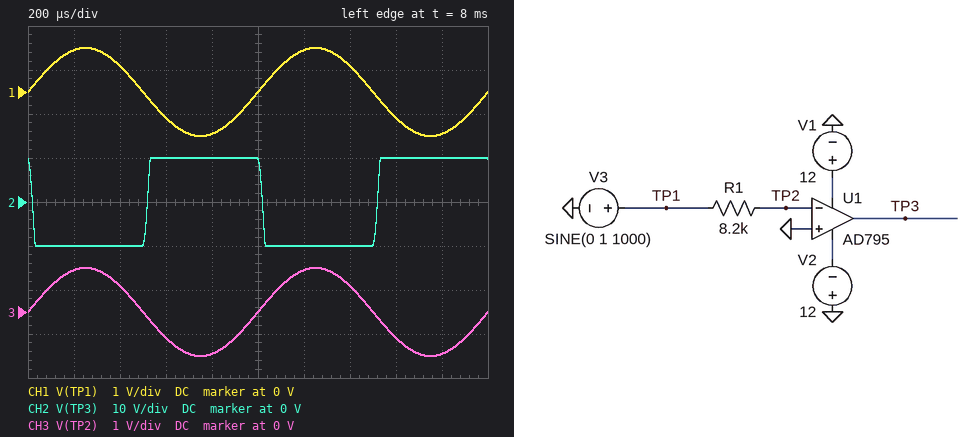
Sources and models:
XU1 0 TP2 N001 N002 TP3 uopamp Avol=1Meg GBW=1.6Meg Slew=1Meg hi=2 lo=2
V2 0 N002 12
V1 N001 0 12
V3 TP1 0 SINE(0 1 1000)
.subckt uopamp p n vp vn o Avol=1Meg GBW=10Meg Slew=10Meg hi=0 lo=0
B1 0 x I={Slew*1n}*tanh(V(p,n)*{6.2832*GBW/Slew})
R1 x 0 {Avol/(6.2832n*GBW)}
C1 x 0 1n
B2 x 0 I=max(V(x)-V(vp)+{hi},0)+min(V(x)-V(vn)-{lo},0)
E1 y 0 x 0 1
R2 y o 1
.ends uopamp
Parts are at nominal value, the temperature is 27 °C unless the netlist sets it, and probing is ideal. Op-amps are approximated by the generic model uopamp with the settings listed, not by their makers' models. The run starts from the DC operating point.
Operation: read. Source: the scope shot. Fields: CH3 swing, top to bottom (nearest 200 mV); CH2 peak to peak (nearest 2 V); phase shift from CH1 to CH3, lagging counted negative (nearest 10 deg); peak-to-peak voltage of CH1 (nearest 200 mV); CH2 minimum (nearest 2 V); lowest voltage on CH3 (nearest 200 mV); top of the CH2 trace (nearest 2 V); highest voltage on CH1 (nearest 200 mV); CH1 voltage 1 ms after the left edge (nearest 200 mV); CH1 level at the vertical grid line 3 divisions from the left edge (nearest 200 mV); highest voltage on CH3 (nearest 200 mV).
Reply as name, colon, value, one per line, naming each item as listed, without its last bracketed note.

CH3 swing, top to bottom: 2.0 V
CH2 peak to peak: 20 V
phase shift from CH1 to CH3, lagging counted negative: 0 deg
peak-to-peak voltage of CH1: 2.0 V
CH2 minimum: -10 V
lowest voltage on CH3: -1.0 V
top of the CH2 trace: 10 V
highest voltage on CH1: 1.0 V
CH1 voltage 1 ms after the left edge: 0 V
CH1 level at the vertical grid line 3 divisions from the left edge: -600 mV
highest voltage on CH3: 1.0 V
